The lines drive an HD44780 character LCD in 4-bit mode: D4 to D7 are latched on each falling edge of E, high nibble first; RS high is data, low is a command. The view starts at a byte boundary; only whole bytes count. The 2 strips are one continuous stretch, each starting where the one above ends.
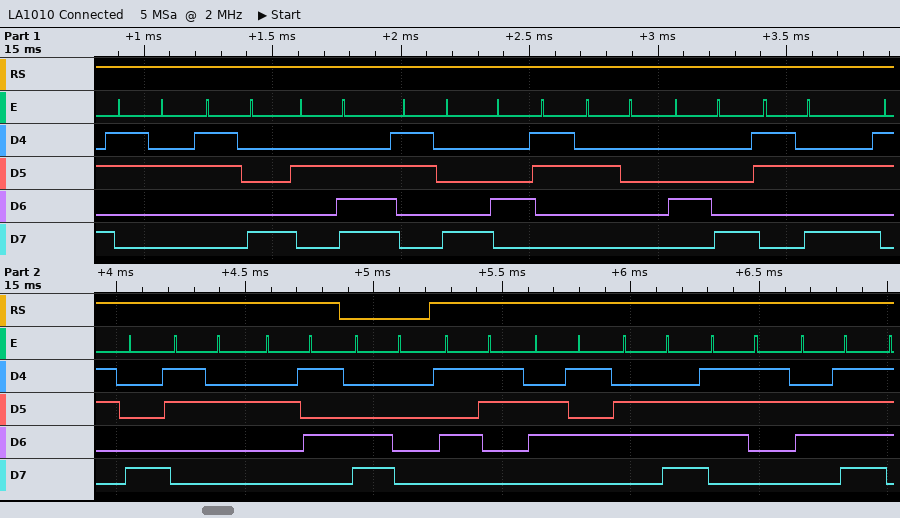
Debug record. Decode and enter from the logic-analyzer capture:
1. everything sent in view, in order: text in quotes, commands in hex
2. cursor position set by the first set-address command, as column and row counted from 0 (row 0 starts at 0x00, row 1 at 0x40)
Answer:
"28.8C H:82%" 0xC0 "Senso"
column 0, row 1
